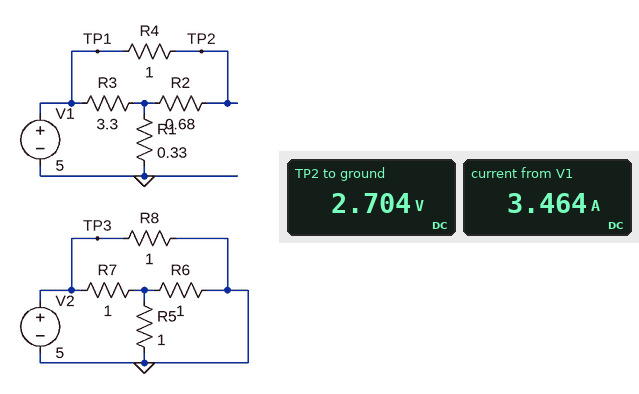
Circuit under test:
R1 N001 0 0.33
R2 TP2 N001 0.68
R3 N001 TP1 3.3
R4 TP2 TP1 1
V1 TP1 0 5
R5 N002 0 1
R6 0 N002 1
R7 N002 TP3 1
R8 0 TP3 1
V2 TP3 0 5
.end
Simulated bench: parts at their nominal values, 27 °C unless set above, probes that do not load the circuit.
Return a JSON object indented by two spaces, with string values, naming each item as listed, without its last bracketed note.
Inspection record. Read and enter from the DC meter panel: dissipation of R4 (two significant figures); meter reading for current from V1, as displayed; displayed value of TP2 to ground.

{
  "dissipation of R4": "5.3 W",
  "meter reading for current from V1, as displayed": "3.464 A",
  "displayed value of TP2 to ground": "2.704 V"
}
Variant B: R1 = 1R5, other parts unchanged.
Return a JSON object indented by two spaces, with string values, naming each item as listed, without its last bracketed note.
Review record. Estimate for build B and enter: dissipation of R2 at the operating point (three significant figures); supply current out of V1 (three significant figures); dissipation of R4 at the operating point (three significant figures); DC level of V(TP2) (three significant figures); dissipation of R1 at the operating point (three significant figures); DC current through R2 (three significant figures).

{
  "dissipation of R2 at the operating point": "1.09 W",
  "supply current out of V1": "1.91 A",
  "dissipation of R4 at the operating point": "1.61 W",
  "DC level of V(TP2)": "3.73 V",
  "dissipation of R1 at the operating point": "5.49 W",
  "DC current through R2": "1.27 A"
}
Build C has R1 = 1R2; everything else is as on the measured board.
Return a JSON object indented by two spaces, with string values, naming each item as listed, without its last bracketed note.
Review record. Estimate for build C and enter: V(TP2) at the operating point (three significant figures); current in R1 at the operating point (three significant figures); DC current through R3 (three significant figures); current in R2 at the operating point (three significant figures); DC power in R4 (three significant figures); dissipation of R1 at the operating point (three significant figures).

{
  "V(TP2) at the operating point": "3.57 V",
  "current in R1 at the operating point": "2.16 A",
  "DC current through R3": "729 mA",
  "current in R2 at the operating point": "1.43 A",
  "DC power in R4": "2.05 W",
  "dissipation of R1 at the operating point": "5.61 W"
}
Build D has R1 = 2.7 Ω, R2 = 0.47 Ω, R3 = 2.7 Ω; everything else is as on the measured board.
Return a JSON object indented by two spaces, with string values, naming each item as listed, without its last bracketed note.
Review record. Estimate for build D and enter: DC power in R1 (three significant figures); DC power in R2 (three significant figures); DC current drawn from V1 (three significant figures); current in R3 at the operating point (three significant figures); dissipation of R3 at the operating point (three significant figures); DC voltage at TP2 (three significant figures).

{
  "DC power in R1": "5.06 W",
  "DC power in R2": "369 mW",
  "DC current drawn from V1": "1.37 A",
  "current in R3 at the operating point": "483 mA",
  "dissipation of R3 at the operating point": "629 mW",
  "DC voltage at TP2": "4.11 V"
}
